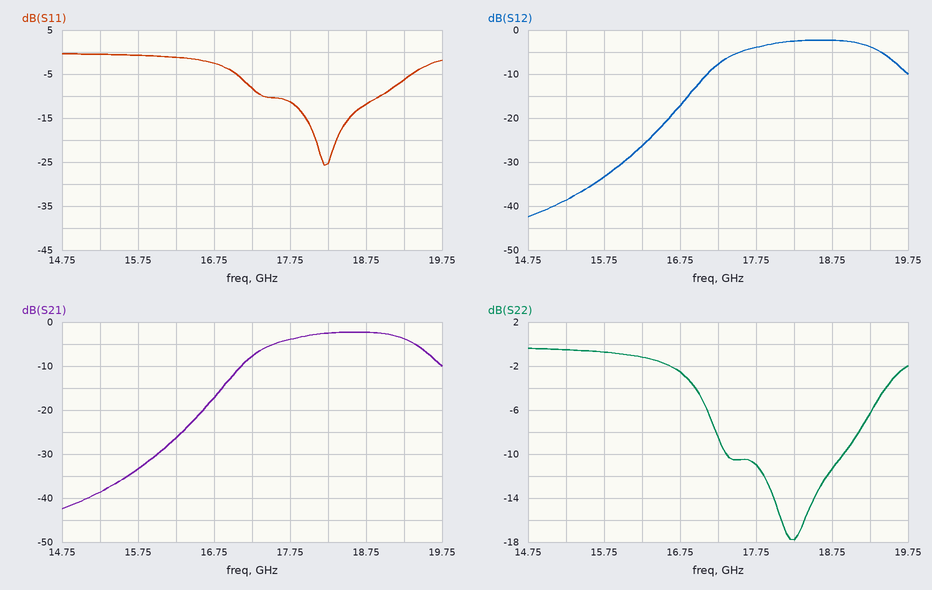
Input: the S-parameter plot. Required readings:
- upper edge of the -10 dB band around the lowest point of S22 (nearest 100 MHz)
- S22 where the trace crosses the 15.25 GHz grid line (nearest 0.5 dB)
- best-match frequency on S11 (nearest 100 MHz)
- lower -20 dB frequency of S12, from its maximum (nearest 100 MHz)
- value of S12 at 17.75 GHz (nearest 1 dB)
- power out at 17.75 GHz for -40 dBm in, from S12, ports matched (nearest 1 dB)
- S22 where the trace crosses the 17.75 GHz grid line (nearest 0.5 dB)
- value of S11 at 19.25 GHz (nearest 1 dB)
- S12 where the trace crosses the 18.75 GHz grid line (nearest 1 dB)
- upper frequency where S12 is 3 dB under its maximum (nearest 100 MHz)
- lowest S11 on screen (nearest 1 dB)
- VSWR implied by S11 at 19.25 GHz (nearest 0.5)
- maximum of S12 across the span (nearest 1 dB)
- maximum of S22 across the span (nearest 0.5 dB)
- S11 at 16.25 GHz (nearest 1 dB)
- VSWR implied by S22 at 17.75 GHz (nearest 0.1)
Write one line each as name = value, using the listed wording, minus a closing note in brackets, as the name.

upper edge of the -10 dB band around the lowest point of S22 = 18.9 GHz
S22 where the trace crosses the 15.25 GHz grid line = -0.5 dB
best-match frequency on S11 = 18.2 GHz
lower -20 dB frequency of S12, from its maximum = 16.5 GHz
value of S12 at 17.75 GHz = -4 dB
power out at 17.75 GHz for -40 dBm in, from S12, ports matched = -44 dBm
S22 where the trace crosses the 17.75 GHz grid line = -11.0 dB
value of S11 at 19.25 GHz = -6 dB
S12 where the trace crosses the 18.75 GHz grid line = -2 dB
upper frequency where S12 is 3 dB under its maximum = 19.4 GHz
lowest S11 on screen = -26 dB
VSWR implied by S11 at 19.25 GHz = 3.0
maximum of S12 across the span = -2 dB
maximum of S22 across the span = -0.5 dB
S11 at 16.25 GHz = -1 dB
VSWR implied by S22 at 17.75 GHz = 1.8
